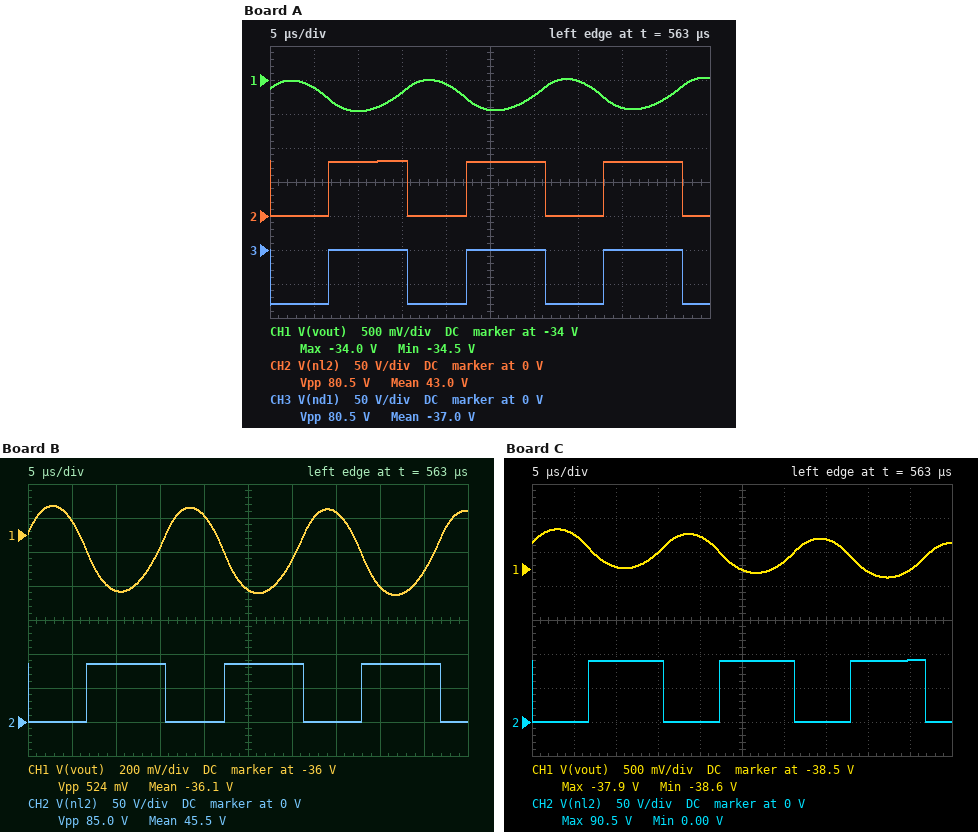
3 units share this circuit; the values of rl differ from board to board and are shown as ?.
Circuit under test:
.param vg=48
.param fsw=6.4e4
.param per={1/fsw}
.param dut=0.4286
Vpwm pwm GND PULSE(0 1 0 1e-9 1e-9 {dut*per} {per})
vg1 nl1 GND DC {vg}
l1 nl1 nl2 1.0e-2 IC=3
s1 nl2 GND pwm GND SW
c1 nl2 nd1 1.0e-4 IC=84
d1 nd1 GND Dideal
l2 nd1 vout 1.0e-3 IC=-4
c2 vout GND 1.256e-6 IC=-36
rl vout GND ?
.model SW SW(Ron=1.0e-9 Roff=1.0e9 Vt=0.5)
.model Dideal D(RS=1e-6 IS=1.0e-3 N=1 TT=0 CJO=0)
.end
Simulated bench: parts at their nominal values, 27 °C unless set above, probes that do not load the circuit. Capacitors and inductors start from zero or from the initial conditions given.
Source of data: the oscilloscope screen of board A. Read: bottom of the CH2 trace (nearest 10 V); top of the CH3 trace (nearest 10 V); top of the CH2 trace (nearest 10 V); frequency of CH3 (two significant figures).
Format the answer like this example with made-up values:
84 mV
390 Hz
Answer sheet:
0 V
0 V
80 V
64 kHz
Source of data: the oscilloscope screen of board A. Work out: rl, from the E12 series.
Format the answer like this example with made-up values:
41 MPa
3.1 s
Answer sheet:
5.6 Ω
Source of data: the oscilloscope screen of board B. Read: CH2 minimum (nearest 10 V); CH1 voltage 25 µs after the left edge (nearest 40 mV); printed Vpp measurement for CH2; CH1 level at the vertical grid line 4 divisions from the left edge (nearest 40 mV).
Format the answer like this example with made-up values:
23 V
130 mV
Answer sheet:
0 V
-36.32 V
85.0 V
-35.88 V
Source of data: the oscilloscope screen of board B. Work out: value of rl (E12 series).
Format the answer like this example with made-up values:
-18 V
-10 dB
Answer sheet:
10 Ω
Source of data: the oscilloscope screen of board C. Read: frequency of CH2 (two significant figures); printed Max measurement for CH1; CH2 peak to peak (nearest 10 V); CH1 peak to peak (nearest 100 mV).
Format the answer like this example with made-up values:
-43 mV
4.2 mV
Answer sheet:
64 kHz
-37.9 V
90 V
700 mV
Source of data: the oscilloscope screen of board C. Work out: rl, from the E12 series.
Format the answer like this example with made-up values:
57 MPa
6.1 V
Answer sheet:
27 Ω
